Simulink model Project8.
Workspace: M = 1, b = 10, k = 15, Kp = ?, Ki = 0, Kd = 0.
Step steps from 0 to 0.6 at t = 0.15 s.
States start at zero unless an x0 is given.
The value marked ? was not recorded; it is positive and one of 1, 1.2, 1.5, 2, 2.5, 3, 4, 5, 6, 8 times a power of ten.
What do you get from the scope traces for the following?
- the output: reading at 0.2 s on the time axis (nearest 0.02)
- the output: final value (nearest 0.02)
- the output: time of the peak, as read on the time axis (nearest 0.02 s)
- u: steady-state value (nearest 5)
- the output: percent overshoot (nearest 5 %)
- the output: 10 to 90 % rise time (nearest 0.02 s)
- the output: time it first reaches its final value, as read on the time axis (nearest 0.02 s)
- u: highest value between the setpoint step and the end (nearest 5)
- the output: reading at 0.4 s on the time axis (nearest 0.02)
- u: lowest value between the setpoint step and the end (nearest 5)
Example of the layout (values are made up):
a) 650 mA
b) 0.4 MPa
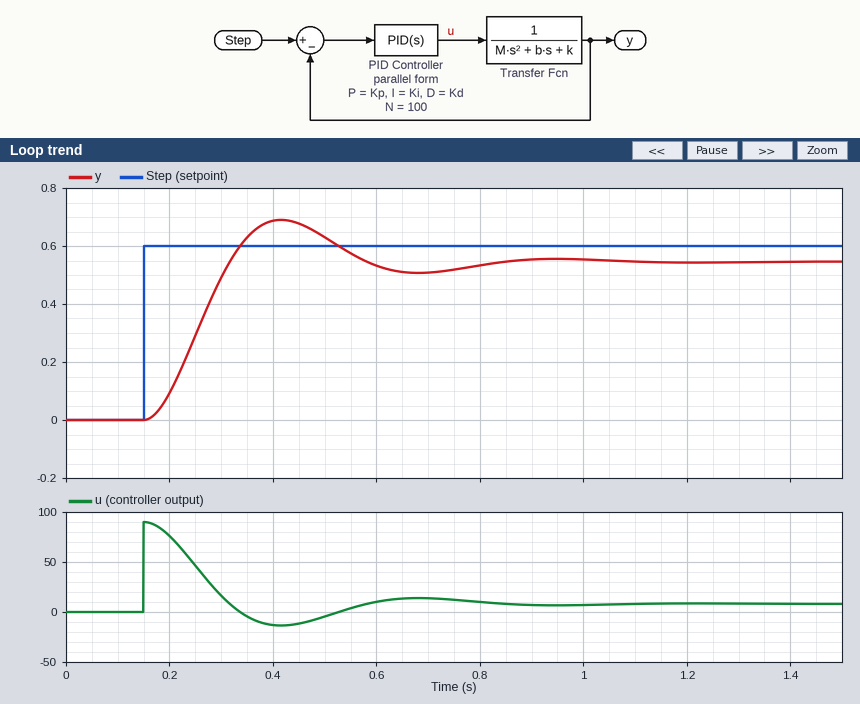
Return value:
a) 0.10
b) 0.54
c) 0.42 s
d) 10
e) 25 %
f) 0.12 s
g) 0.32 s
h) 90
i) 0.68
j) -15
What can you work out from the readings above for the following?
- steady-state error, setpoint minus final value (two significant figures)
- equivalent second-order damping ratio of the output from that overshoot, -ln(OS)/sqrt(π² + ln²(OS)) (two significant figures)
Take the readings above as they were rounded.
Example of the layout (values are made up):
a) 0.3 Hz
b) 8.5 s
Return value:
a) 0.060
b) 0.40
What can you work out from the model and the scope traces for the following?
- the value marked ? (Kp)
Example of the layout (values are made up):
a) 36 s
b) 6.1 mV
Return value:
a) 150
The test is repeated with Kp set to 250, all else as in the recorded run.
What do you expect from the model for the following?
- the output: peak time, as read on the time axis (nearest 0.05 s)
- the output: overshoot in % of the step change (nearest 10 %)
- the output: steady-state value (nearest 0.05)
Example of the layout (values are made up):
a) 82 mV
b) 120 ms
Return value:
a) 0.35 s
b) 40 %
c) 0.55
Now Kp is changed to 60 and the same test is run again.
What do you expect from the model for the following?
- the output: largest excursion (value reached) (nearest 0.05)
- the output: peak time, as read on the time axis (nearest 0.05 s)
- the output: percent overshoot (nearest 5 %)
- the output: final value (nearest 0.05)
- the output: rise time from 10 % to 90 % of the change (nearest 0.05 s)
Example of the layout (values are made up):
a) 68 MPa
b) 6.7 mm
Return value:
a) 0.55
b) 0.60 s
c) 10 %
d) 0.50
e) 0.20 s
